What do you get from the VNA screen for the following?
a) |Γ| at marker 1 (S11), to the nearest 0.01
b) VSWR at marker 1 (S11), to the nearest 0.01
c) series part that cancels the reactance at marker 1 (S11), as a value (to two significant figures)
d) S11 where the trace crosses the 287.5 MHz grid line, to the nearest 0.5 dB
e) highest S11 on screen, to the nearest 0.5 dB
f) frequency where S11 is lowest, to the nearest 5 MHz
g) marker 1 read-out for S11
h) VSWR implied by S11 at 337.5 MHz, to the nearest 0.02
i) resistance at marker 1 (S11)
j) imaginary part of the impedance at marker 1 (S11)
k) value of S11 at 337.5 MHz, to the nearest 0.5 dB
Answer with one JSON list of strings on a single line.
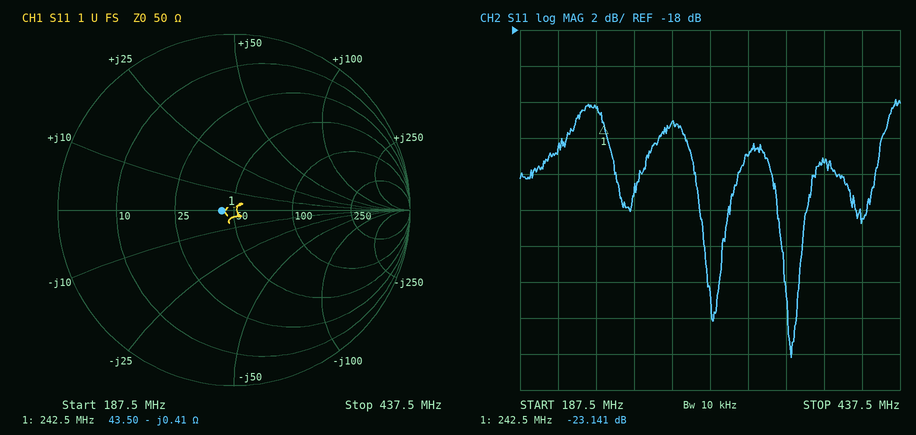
["0.07", "1.15", "270 pH", "-23.0 dB", "-22.0 dB", "365 MHz", "-23.141 dB", "1.12", "43.50 Ω", "-0.41 Ω", "-25.0 dB"]
